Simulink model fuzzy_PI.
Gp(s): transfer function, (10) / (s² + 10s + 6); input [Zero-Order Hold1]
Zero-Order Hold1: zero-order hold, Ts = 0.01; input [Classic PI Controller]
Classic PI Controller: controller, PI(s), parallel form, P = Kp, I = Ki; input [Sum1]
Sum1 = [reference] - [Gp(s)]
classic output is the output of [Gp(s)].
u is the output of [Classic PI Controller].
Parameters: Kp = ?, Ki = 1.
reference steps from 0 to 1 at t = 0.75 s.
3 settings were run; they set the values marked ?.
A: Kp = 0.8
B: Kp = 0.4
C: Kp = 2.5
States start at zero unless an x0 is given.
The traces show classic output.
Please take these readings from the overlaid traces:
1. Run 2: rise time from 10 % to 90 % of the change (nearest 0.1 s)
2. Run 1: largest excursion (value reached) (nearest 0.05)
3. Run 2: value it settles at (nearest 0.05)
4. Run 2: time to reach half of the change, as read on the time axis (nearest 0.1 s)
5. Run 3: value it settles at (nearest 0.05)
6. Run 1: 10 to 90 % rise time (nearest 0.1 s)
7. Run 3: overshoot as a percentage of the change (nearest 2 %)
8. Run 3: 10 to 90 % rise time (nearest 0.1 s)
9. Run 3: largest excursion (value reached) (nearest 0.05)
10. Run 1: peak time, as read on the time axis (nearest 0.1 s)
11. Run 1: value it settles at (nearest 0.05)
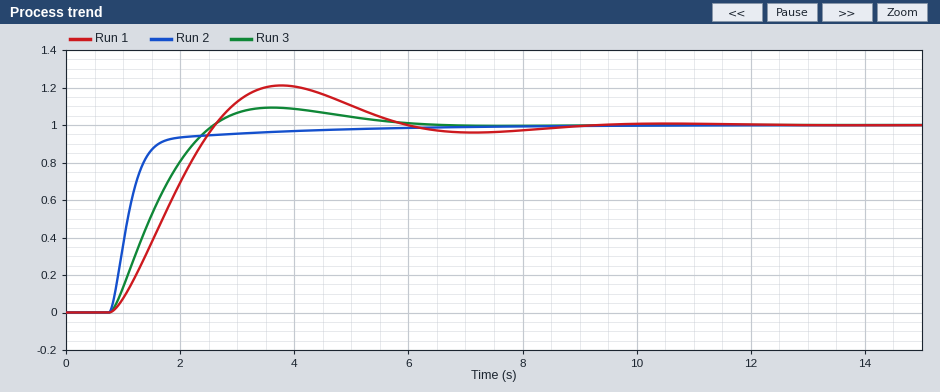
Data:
0.8 s
1.20
1.00
1.1 s
1.00
1.3 s
10 %
1.3 s
1.10
3.8 s
1.00
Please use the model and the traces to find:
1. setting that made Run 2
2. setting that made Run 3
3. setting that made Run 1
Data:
C
A
B
